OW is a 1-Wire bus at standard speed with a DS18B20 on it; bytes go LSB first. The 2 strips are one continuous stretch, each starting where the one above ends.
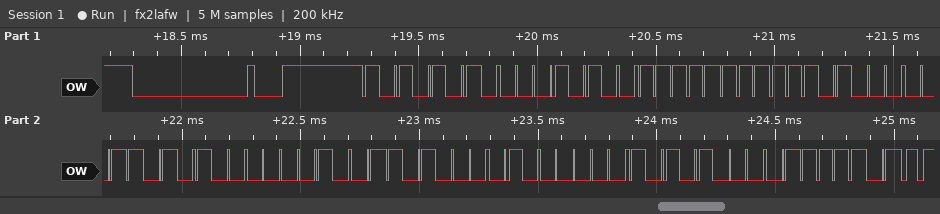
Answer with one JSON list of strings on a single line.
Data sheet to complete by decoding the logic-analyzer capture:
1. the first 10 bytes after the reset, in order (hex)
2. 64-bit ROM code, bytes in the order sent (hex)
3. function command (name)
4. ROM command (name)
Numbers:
["55 28 FF 17 AC 40 16 02 15 BE", "28 FF 17 AC 40 16 02 15", "Read Scratchpad", "Match ROM"]
